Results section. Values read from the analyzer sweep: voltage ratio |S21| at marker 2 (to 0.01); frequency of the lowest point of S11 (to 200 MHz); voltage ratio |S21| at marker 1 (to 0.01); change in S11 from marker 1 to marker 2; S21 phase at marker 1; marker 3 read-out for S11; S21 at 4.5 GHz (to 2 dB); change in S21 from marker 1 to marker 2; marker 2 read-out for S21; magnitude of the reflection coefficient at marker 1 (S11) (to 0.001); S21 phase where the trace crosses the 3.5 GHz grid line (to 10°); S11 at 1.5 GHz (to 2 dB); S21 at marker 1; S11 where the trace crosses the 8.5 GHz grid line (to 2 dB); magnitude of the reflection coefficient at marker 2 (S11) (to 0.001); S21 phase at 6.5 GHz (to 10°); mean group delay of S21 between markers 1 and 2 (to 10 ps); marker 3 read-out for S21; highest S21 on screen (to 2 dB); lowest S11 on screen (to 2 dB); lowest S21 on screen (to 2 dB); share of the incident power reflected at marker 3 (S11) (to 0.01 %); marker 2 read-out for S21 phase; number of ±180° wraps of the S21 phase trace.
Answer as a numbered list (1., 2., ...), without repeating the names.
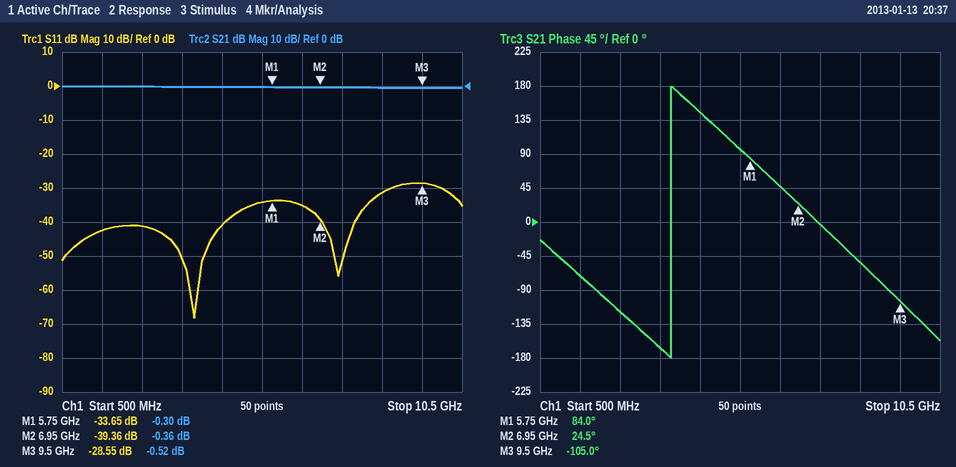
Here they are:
1. 0.96
2. 3.8 GHz
3. 0.97
4. -5.71 dB
5. 84.0°
6. -28.55 dB
7. 0 dB
8. -0.06 dB
9. -0.36 dB
10. 0.021
11. -170°
12. -42 dB
13. -0.30 dB
14. -32 dB
15. 0.011
16. 50°
17. 140 ps
18. -0.52 dB
19. 0 dB
20. -68 dB
21. 0 dB
22. 0.14 %
23. 24.5°
24. 1
